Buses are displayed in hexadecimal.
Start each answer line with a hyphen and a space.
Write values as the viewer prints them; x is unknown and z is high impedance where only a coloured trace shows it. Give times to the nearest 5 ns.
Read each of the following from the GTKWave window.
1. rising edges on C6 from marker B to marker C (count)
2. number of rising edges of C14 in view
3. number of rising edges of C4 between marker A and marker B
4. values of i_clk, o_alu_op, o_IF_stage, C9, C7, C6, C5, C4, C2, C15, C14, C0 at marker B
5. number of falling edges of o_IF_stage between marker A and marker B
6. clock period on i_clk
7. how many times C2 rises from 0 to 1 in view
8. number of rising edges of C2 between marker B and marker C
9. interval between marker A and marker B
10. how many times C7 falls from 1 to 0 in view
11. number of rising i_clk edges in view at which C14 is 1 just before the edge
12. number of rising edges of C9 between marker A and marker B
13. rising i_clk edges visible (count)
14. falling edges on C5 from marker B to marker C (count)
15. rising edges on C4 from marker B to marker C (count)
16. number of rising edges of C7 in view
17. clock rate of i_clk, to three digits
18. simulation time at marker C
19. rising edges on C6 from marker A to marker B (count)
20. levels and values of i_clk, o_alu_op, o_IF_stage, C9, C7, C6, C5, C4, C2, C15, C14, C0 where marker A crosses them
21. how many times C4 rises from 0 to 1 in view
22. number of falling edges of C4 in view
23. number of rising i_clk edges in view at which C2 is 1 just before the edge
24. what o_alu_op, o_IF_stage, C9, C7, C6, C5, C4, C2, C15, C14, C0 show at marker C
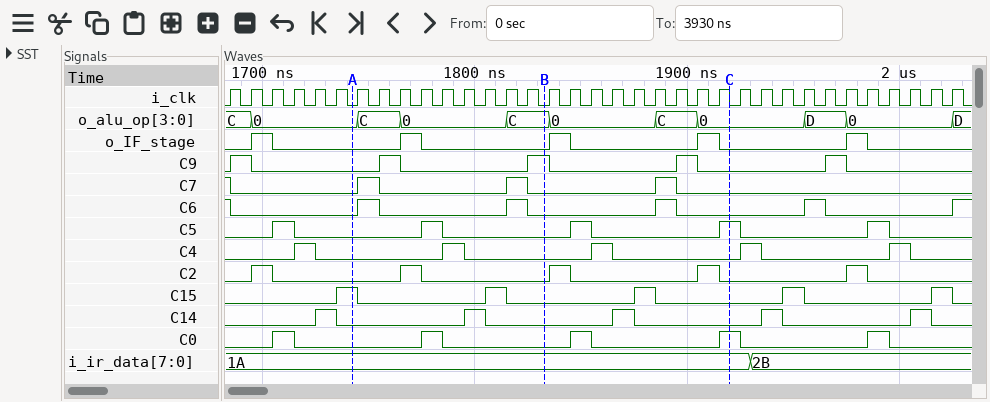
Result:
- 1
- 5
- 1
- i_clk=0, o_alu_op=C, o_IF_stage=0, C9=1, C7=0, C6=0, C5=0, C4=0, C2=0, C15=0, C14=0, C0=0
- 1
- 10 ns
- 5
- 2
- 90 ns
- 4
- 5
- 2
- 35
- 1
- 1
- 3
- 100 MHz
- 1920 ns
- 2
- i_clk=0, o_alu_op=0, o_IF_stage=0, C9=0, C7=0, C6=0, C5=0, C4=0, C2=0, C15=1, C14=0, C0=0
- 5
- 5
- 5
- o_alu_op=0, o_IF_stage=0, C9=0, C7=0, C6=0, C5=1, C4=0, C2=0, C15=0, C14=0, C0=1
